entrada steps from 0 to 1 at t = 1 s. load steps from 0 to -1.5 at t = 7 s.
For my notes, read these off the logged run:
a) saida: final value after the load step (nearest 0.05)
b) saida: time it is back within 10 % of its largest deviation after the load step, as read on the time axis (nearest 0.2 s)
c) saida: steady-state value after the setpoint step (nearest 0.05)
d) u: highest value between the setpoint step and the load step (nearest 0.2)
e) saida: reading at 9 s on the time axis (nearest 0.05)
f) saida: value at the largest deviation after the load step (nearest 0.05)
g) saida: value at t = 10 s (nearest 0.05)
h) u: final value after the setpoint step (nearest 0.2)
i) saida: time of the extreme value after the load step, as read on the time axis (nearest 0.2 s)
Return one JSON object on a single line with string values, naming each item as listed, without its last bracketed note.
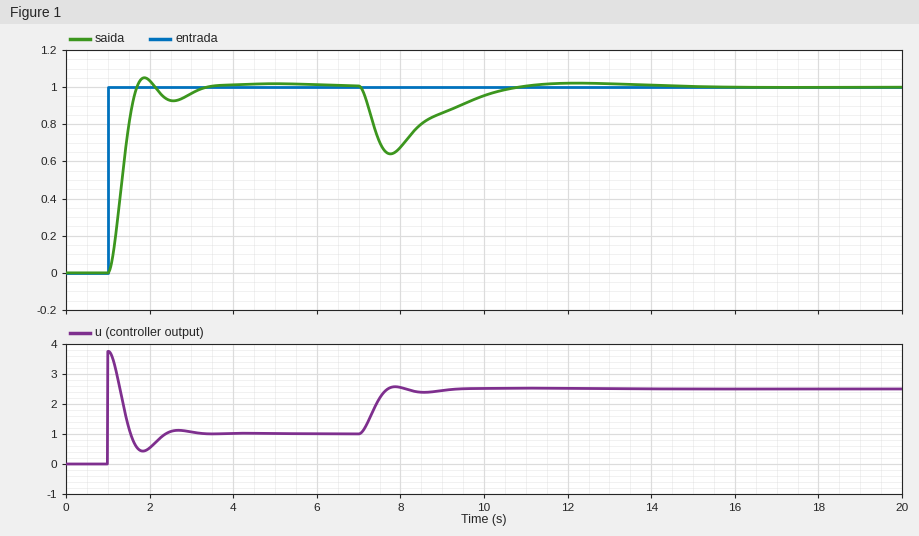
{"saida: final value after the load step": "1.00", "saida: time it is back within 10 % of its largest deviation after the load step, as read on the time axis": "10.2 s", "saida: steady-state value after the setpoint step": "1.00", "u: highest value between the setpoint step and the load step": "3.8", "saida: reading at 9 s on the time axis": "0.85", "saida: value at the largest deviation after the load step": "0.65", "saida: value at t = 10 s": "0.95", "u: final value after the setpoint step": "1.0", "saida: time of the extreme value after the load step, as read on the time axis": "7.8 s"}
